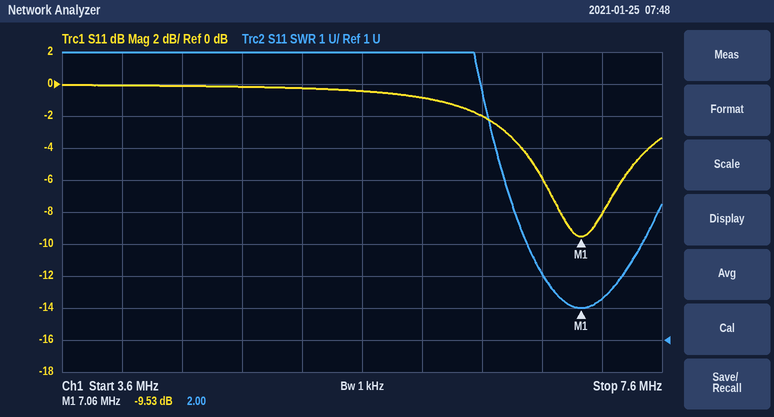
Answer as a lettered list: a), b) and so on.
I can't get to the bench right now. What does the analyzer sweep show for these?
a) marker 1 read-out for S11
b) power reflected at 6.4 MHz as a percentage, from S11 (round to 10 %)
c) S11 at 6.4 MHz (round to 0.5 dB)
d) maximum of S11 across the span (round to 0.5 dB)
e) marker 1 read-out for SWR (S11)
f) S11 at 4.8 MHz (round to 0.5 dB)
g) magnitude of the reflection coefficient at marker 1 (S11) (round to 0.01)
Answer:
a) -9.53 dB
b) 60 %
c) -2.0 dB
d) 0.0 dB
e) 2.00
f) 0.0 dB
g) 0.33
